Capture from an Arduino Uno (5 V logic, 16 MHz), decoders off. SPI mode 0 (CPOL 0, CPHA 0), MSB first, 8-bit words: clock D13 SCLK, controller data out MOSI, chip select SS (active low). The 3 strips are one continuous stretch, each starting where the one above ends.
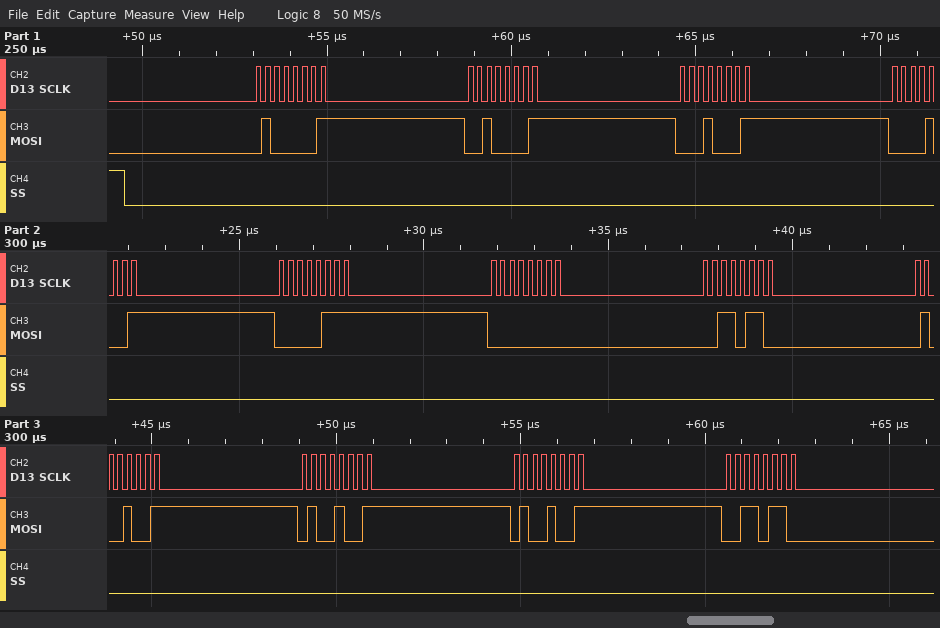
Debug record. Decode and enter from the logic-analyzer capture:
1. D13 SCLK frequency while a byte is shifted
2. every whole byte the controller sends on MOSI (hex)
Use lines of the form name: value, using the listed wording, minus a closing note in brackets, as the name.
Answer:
D13 SCLK frequency while a byte is shifted: 4 MHz
every whole byte the controller sends on MOSI: 41 21 11 09 07 00 36 49 49 49 36
